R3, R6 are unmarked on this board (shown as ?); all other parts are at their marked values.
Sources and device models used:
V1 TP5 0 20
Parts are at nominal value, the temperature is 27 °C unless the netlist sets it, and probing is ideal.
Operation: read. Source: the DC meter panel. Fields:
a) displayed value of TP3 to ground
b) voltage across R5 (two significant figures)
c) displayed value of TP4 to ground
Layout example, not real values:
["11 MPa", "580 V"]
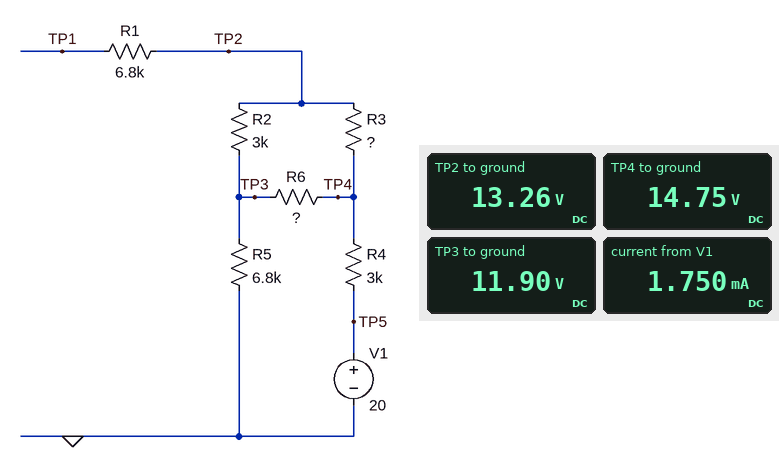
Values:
["11.90 V", "12 V", "14.75 V"]
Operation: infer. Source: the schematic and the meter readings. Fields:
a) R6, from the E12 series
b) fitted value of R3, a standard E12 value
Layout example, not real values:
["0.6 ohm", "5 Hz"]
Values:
["2.2 kΩ", "3.3 kΩ"]
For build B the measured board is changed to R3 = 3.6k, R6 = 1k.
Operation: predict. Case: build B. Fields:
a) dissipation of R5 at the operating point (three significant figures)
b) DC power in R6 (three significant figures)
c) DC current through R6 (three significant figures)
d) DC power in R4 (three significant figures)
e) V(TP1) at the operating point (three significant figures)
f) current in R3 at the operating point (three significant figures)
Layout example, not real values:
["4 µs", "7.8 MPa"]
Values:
["23.9 mW", "2.65 mW", "1.63 mA", "10.5 mW", "13.5 V", "247 µA"]
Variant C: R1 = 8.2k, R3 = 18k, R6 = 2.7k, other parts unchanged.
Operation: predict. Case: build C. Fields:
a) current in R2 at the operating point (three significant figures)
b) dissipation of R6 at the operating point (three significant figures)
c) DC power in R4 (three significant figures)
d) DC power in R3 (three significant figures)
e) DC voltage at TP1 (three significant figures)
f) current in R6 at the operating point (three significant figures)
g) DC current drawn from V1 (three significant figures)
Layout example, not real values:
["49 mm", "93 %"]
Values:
["187 µA", "5.70 mW", "8.07 mW", "629 µW", "11.7 V", "1.45 mA", "1.64 mA"]
